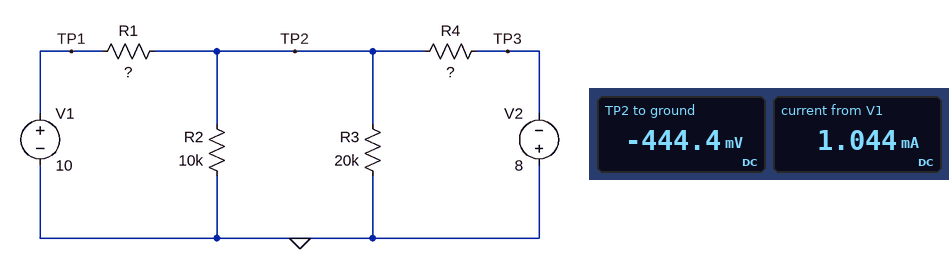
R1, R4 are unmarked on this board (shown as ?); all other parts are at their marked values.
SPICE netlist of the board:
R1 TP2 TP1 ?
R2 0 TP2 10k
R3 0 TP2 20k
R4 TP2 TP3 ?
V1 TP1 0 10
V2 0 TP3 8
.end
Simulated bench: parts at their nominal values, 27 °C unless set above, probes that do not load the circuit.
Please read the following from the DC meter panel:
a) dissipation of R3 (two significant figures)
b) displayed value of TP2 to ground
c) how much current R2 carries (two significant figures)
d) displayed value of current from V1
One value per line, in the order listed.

9.9 µW
-444.4 mV
44 µA
1.044 mA
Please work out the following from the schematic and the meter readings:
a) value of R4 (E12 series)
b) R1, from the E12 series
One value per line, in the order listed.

6.8 kΩ
10 kΩ
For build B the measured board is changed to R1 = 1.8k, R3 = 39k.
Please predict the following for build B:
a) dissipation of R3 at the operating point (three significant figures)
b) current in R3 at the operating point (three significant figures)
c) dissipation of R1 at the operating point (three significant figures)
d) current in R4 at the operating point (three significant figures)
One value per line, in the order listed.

717 µW
136 µA
12.3 mW
1.95 mA
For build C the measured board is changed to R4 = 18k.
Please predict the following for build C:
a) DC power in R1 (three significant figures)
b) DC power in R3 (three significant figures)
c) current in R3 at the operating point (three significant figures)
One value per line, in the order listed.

6.69 mW
165 µW
90.9 µA
